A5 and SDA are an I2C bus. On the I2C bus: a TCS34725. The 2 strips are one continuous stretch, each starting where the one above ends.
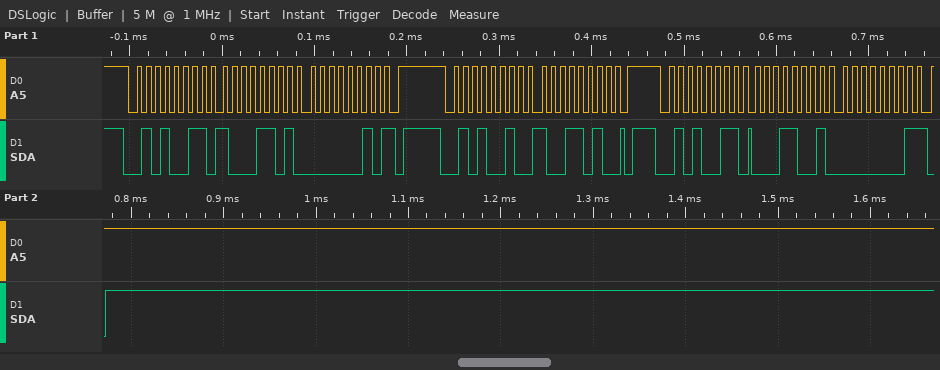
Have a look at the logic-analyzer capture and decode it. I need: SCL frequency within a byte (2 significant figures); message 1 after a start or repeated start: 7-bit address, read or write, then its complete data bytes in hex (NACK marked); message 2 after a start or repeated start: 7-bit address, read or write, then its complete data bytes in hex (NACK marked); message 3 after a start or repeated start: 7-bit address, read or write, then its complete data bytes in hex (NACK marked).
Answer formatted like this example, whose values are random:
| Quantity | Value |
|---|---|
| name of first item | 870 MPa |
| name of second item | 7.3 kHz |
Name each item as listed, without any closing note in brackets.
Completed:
| Quantity | Value |
|---|---|
| SCL frequency within a byte | 100 kHz |
| message 1 after a start or repeated start: 7-bit address, read or write, then its complete data bytes in hex | 0x29 read: 8D 02 NACK |
| message 2 after a start or repeated start: 7-bit address, read or write, then its complete data bytes in hex | 0x29 write: 9A |
| message 3 after a start or repeated start: 7-bit address, read or write, then its complete data bytes in hex | 0x29 read: 19 01 NACK |
